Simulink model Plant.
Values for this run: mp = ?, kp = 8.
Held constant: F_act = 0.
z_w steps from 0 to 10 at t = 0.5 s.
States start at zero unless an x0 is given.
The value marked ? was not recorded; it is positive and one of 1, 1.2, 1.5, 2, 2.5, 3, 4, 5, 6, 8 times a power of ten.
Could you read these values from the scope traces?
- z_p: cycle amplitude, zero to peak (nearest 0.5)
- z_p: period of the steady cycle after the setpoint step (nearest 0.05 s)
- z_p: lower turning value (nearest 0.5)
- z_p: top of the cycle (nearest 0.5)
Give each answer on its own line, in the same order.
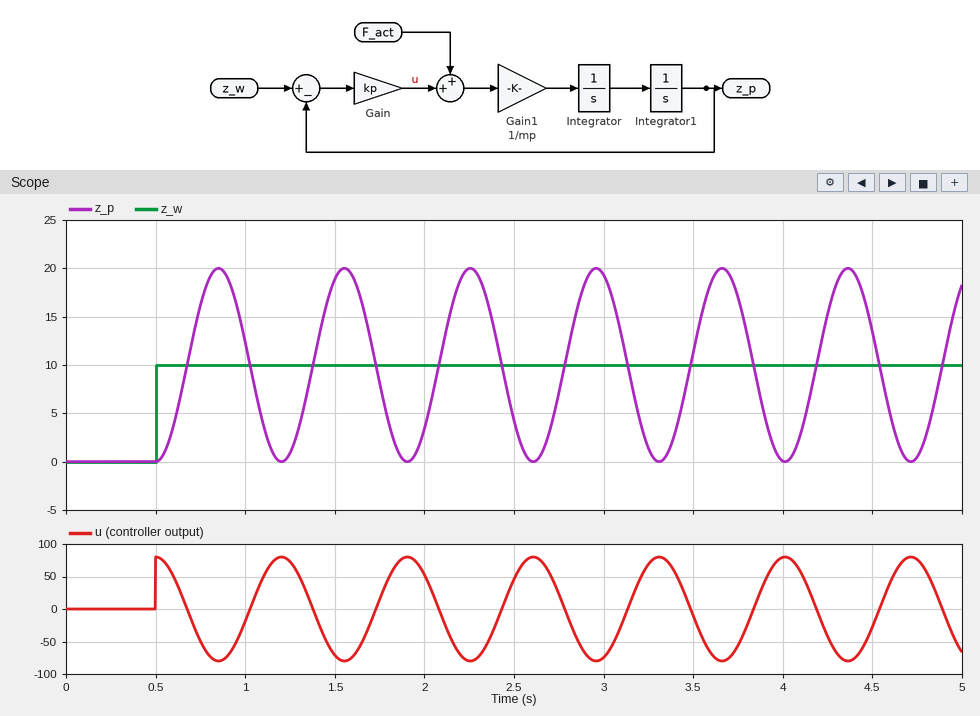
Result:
10.0
0.70 s
0.0
20.0
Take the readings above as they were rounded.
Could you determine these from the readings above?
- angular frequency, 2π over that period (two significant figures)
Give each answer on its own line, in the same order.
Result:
9.0 rad/s
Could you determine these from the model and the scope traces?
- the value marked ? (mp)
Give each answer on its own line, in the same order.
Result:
0.1
